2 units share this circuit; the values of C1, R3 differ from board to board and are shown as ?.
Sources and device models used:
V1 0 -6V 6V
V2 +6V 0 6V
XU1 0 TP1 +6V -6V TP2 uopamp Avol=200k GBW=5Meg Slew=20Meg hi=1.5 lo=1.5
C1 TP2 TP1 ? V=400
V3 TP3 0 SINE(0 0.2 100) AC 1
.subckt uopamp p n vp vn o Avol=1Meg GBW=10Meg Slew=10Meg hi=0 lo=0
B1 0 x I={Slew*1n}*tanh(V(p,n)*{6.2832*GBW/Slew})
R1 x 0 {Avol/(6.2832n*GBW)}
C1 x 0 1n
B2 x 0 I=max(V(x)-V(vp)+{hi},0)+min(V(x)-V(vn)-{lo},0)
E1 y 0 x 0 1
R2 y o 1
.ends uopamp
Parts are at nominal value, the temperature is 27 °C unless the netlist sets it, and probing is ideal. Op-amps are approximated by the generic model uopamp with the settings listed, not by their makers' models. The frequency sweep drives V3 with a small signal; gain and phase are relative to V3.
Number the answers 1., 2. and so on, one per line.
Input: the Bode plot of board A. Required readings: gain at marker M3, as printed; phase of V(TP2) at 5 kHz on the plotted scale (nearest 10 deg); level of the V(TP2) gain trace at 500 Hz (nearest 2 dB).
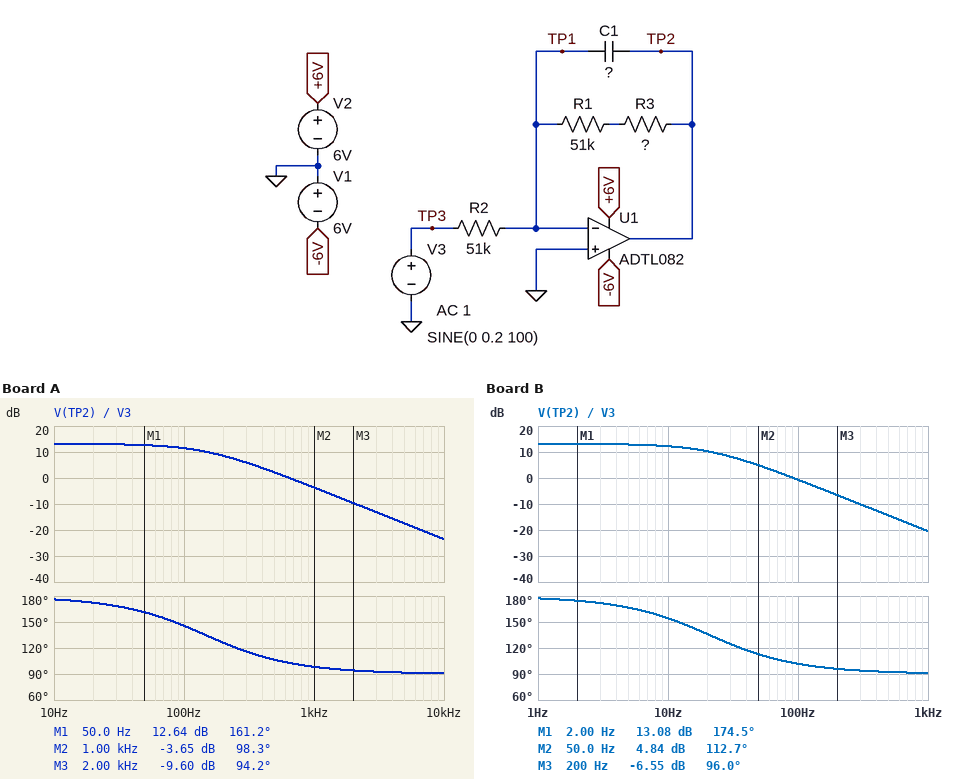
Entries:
1. -9.60 dB
2. 90 deg
3. 2 dB
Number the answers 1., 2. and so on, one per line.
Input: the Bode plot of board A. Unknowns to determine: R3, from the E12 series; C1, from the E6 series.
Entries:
1. 180 kΩ
2. 4.7 nF
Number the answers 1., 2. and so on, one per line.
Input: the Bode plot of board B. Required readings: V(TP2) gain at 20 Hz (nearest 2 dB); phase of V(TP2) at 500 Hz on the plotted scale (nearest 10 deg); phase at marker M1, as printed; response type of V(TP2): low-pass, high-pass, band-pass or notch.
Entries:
1. 10 dB
2. 90 deg
3. 174.5 deg
4. low-pass
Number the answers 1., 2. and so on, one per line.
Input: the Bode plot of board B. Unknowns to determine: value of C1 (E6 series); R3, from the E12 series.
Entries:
1. 33 nF
2. 180 kΩ
